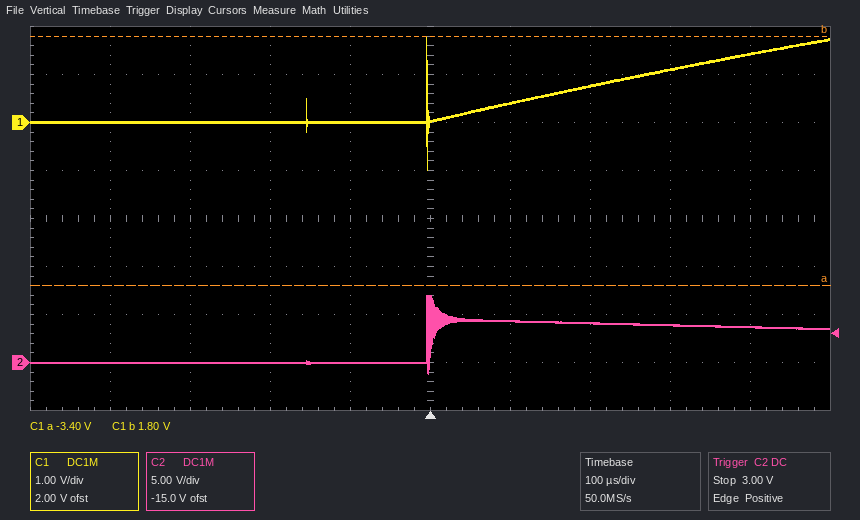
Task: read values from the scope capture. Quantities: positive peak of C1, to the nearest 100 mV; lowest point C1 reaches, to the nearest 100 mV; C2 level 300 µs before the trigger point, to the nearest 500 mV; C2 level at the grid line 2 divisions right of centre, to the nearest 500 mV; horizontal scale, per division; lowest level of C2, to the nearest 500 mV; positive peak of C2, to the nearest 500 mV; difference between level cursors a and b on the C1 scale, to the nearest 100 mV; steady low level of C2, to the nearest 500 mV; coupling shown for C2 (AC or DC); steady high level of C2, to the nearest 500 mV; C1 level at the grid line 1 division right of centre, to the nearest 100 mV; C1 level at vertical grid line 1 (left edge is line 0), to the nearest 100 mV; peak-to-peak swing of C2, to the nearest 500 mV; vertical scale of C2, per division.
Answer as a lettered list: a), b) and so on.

a) 1.8 V
b) -1.0 V
c) 0.0 V
d) 4.0 V
e) 100 µs
f) -1.0 V
g) 7.0 V
h) 5.2 V
i) 0.0 V
j) DC
k) 4.0 V
l) 400 mV
m) 0.0 V
n) 8.0 V
o) 5 V
